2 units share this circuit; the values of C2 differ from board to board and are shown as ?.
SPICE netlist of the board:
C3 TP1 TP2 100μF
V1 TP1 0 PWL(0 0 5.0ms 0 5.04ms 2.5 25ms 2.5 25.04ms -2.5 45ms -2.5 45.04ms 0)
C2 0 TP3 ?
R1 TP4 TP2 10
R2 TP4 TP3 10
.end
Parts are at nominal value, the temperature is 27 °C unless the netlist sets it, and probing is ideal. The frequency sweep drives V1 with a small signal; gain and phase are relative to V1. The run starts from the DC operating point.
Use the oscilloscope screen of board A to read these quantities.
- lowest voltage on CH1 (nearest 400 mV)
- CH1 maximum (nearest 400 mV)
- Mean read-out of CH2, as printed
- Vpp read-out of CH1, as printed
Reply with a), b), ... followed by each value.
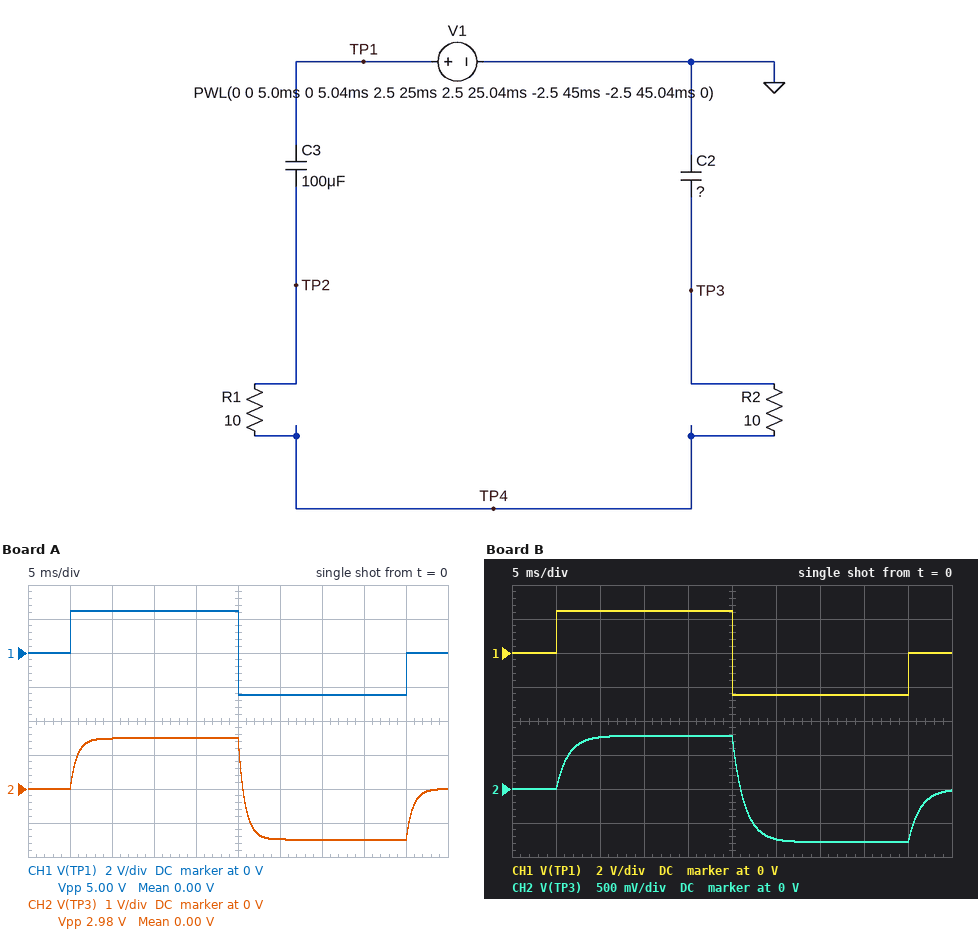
a) -2.4 V
b) 2.4 V
c) 0.00 V
d) 5.00 V
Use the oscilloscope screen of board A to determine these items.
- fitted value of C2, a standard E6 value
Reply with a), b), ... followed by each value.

a) 68 µF
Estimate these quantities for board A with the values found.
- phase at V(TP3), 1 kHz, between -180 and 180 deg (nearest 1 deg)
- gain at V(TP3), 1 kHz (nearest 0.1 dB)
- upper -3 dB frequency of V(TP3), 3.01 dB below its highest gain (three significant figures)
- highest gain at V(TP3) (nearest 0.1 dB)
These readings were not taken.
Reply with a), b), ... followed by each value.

a) -79 deg
b) -18.8 dB
c) 197 Hz
d) -4.5 dB
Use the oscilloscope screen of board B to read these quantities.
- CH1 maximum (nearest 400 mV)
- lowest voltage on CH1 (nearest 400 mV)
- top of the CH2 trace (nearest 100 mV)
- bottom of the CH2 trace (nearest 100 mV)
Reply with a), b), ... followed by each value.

a) 2.4 V
b) -2.4 V
c) 800 mV
d) -800 mV
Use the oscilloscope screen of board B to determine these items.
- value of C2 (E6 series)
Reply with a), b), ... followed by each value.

a) 220 µF
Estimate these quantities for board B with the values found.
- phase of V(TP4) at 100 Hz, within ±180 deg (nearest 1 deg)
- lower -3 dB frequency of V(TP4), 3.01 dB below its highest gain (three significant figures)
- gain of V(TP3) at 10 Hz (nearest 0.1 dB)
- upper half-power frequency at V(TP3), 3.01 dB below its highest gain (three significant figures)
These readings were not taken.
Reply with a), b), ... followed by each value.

a) 13 deg
b) 54.1 Hz
c) -10.1 dB
d) 116 Hz
